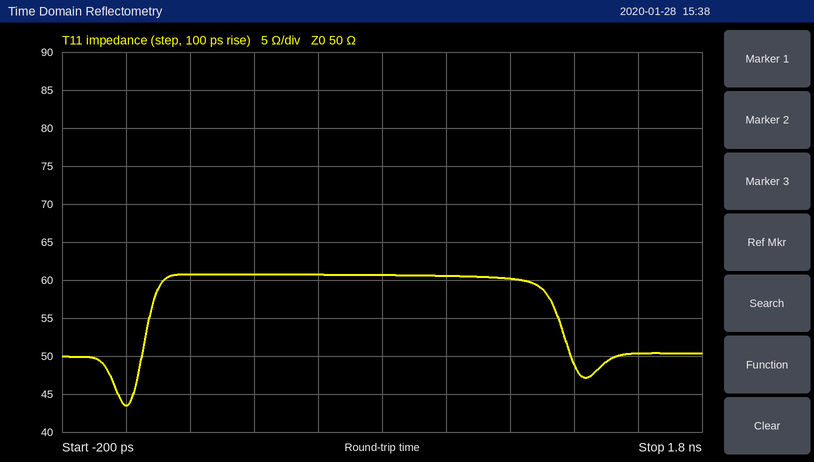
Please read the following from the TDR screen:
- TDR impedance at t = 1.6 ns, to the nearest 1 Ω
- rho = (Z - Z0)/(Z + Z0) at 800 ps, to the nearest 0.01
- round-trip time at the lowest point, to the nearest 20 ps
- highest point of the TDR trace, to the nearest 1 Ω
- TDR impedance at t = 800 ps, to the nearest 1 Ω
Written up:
50 Ω
+0.10
0 ps
61 Ω
61 Ω
